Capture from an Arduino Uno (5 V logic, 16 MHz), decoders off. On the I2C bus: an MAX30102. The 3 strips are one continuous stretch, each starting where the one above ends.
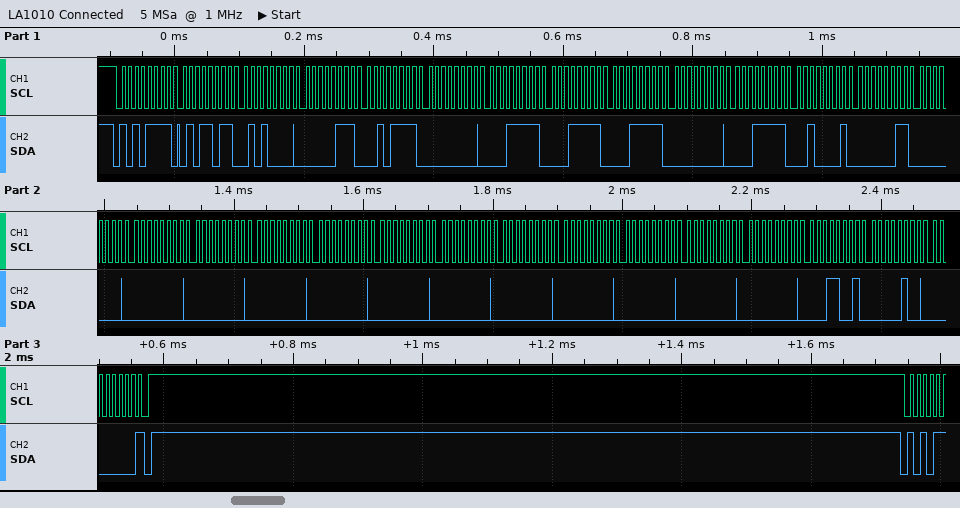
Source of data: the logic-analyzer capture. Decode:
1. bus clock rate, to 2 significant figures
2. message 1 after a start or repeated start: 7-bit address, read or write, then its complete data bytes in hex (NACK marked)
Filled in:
100 kHz
0x57 read: 5B 50 07 2F 00 1F 1F 1F 00 1F 21 03 00 00 00 00 00 00 00 00 00 00 00 00 19 04 00 NACK
